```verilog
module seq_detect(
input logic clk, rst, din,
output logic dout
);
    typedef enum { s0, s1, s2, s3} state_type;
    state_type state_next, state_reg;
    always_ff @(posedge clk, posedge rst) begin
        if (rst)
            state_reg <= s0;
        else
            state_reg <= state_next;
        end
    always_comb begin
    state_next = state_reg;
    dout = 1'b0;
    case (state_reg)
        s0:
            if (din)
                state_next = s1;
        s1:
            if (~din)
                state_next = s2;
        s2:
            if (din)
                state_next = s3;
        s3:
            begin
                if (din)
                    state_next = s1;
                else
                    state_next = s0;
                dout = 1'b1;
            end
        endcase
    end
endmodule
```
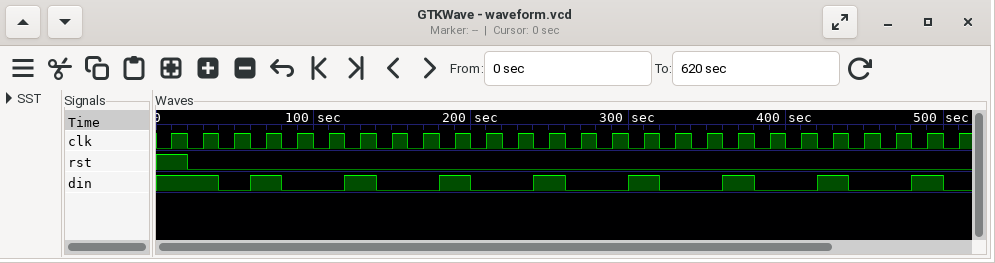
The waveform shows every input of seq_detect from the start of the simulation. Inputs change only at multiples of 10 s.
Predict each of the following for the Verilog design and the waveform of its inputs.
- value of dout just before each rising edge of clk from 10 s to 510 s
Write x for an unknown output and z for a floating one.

0 0 0 0 1 0 0 0 0 0 1 0 0 0 0 0 1 0 0 0 0 0 1 0 0 0
